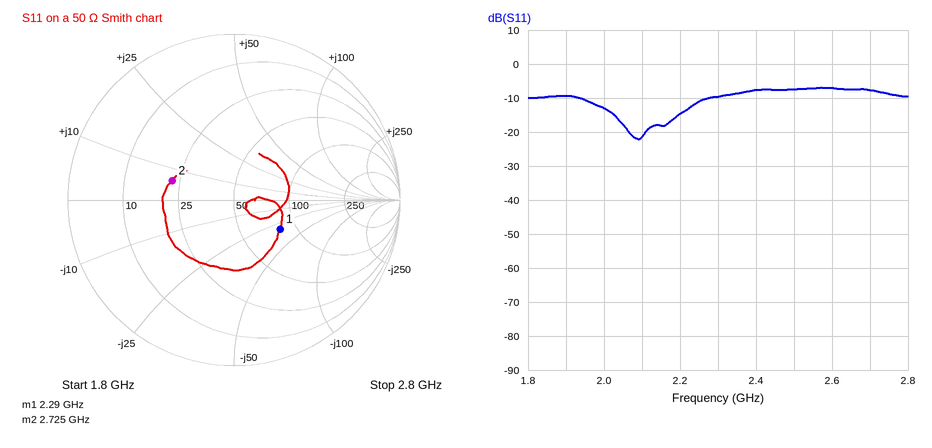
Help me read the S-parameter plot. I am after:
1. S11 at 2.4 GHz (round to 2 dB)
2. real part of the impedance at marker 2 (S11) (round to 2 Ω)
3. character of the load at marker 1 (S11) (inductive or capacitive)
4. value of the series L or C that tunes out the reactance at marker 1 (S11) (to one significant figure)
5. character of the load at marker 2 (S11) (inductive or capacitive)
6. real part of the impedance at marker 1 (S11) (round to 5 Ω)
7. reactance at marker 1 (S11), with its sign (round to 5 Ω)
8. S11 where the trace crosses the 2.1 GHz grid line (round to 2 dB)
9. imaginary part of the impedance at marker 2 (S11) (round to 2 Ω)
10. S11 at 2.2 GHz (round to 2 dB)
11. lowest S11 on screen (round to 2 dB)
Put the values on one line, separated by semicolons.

-8 dB; 22 Ω; capacitive; 2 nH; inductive; 80 Ω; -30 Ω; -22 dB; +6 Ω; -14 dB; -22 dB
